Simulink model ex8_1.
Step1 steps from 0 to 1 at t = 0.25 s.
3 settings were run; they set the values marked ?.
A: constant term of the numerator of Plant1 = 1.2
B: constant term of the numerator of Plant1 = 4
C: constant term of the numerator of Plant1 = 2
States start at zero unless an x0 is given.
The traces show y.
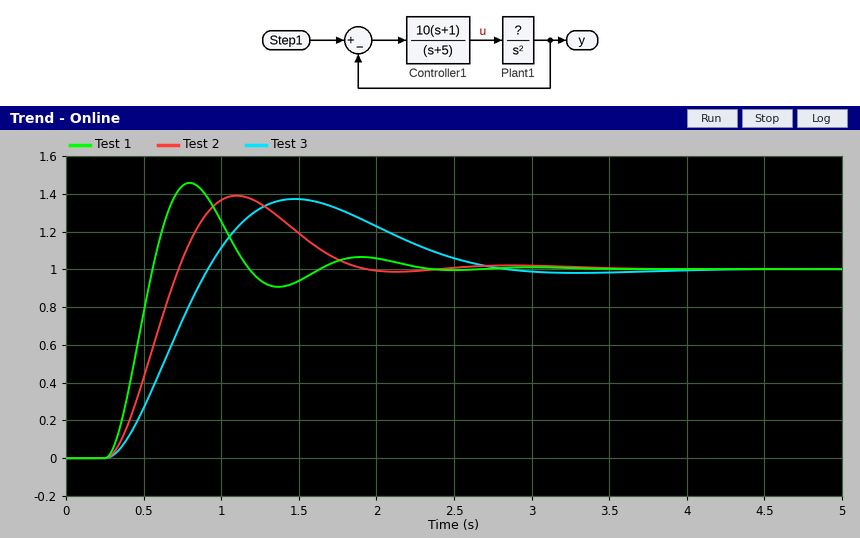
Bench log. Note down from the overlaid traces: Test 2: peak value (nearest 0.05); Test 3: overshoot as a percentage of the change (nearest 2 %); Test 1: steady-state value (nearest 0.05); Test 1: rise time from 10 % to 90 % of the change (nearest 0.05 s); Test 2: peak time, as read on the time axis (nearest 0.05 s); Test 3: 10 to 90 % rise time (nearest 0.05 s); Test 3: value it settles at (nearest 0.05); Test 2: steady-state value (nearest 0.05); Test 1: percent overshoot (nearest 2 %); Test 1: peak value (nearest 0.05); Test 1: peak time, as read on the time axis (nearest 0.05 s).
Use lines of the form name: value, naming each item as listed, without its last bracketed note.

Test 2: peak value: 1.40
Test 3: overshoot as a percentage of the change: 38 %
Test 1: steady-state value: 1.00
Test 1: rise time from 10 % to 90 % of the change: 0.20 s
Test 2: peak time, as read on the time axis: 1.10 s
Test 3: 10 to 90 % rise time: 0.45 s
Test 3: value it settles at: 1.00
Test 2: steady-state value: 1.00
Test 1: percent overshoot: 46 %
Test 1: peak value: 1.45
Test 1: peak time, as read on the time axis: 0.80 s
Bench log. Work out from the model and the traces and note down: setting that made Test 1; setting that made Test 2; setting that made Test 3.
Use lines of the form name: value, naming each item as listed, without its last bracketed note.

setting that made Test 1: B
setting that made Test 2: C
setting that made Test 3: A
